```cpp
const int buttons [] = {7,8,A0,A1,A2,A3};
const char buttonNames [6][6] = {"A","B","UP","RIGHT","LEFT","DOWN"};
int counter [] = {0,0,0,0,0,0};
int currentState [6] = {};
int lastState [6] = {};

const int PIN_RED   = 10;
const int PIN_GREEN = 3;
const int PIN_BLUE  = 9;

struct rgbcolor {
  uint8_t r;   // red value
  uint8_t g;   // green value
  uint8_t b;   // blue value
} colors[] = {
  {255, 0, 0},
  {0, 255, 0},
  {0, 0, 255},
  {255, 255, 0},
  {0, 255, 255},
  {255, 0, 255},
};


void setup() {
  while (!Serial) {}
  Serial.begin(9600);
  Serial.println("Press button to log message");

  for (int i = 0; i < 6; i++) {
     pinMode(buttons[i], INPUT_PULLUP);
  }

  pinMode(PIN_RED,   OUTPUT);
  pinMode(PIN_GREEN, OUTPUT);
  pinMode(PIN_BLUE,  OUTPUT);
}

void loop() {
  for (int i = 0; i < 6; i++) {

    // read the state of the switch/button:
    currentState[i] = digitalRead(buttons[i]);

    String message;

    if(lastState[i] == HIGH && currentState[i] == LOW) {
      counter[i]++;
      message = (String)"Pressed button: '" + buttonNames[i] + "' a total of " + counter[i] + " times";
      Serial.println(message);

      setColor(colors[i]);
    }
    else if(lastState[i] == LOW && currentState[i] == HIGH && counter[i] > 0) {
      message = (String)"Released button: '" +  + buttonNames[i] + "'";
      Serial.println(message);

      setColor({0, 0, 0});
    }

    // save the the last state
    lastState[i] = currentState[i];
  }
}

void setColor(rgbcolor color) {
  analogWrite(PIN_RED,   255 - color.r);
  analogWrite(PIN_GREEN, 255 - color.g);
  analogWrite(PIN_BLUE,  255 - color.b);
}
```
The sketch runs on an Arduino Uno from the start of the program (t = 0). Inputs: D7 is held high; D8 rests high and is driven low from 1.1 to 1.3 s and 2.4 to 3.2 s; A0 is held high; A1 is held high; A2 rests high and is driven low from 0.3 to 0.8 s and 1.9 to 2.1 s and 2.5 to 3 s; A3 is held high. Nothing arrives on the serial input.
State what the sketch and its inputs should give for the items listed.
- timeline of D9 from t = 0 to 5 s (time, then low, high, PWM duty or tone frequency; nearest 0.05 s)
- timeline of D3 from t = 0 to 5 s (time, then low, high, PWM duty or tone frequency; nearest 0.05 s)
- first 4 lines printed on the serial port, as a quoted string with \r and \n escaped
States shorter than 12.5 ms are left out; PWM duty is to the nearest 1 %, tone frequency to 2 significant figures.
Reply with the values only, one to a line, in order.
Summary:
0 s low; 0.8 s high; 1.9 s low; 2.1 s high; 2.5 s low; 3 s high
0 s low; 0.8 s high; 1.1 s low; 1.3 s high; 1.9 s low; 2.1 s high; 2.4 s low; 3 s high
"Press button to log message\r\nPressed button: 'LEFT' a total of 1 times\r\nReleased button: 'LEFT'\r\nPressed button: 'B' a total of 1 times\r\n"
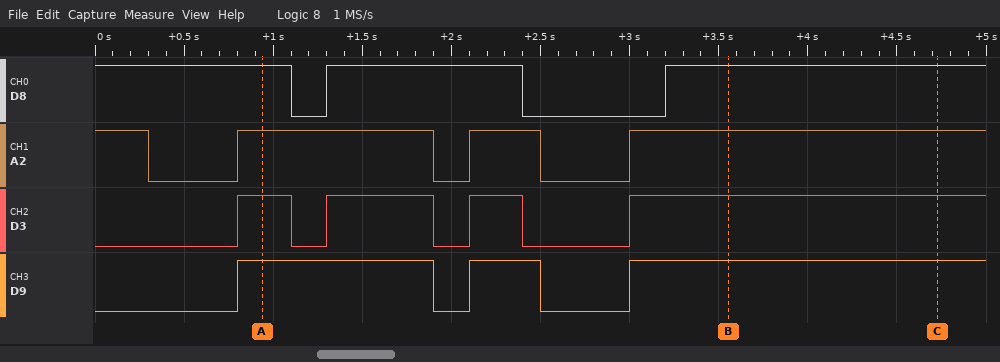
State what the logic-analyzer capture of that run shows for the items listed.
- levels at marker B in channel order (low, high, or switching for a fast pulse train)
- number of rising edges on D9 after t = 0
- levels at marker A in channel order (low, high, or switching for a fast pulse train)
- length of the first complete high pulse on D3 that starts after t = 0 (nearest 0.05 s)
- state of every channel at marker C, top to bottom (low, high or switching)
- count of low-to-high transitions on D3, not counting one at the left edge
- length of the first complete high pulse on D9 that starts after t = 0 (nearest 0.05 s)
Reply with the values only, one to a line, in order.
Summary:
D8 high, A2 high, D3 high, D9 high
3
D8 high, A2 high, D3 high, D9 high
0.30 s
D8 high, A2 high, D3 high, D9 high
4
1.10 s
